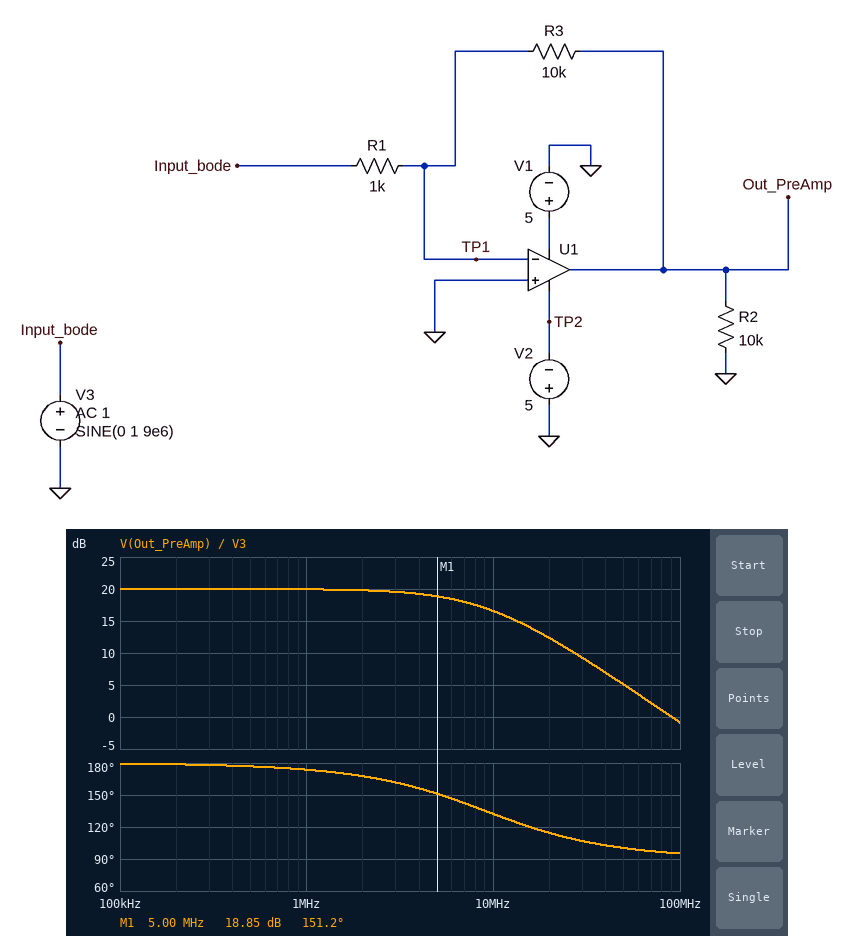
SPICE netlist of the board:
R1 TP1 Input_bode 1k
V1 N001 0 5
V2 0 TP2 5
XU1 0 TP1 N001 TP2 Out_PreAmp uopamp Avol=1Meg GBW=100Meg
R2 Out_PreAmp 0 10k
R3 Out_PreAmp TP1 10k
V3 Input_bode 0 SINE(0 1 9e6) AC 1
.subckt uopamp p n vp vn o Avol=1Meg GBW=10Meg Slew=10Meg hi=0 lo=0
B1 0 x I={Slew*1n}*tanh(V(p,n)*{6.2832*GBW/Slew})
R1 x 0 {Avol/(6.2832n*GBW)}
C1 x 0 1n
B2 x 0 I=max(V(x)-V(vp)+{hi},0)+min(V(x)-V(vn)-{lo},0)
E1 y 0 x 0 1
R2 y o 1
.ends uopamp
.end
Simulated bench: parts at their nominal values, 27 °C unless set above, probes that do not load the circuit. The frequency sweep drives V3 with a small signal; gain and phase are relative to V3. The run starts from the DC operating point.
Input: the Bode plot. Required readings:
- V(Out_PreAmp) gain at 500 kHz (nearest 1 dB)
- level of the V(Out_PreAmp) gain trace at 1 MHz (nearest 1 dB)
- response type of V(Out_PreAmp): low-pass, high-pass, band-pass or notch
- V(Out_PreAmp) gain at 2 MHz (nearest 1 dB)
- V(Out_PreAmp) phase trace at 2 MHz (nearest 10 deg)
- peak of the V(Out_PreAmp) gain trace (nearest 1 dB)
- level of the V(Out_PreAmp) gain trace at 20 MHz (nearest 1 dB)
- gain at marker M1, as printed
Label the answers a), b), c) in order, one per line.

a) 20 dB
b) 20 dB
c) low-pass
d) 20 dB
e) 170 deg
f) 20 dB
g) 12 dB
h) 18.85 dB
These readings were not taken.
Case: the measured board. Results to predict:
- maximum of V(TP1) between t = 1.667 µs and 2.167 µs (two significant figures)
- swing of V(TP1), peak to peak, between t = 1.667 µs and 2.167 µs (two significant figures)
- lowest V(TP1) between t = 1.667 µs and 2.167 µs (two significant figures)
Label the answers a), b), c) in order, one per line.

a) 900 mV
b) 1.8 V
c) -920 mV
